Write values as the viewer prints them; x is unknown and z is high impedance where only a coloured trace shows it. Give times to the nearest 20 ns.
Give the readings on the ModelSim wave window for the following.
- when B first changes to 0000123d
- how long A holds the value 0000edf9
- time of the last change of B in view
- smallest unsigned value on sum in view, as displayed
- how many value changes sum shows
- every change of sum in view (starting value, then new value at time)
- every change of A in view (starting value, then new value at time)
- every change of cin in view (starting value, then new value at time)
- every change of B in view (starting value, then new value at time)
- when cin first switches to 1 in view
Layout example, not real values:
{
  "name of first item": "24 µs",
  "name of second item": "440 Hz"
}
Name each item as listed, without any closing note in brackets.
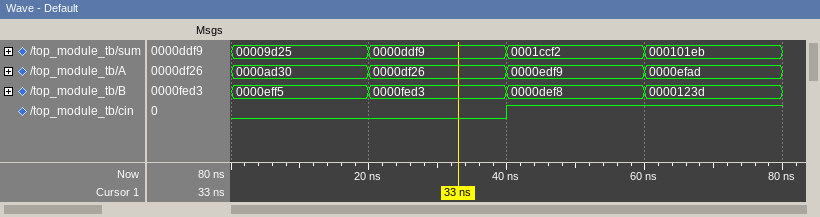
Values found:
{
  "when B first changes to 0000123d": "60 ns",
  "how long A holds the value 0000edf9": "20 ns",
  "time of the last change of B in view": "60 ns",
  "smallest unsigned value on sum in view, as displayed": "00009d25",
  "how many value changes sum shows": "3",
  "every change of sum in view": "00009d25, 0000ddf9 at 20 ns, 0001ccf2 at 40 ns, 000101eb at 60 ns",
  "every change of A in view": "0000ad30, 0000df26 at 20 ns, 0000edf9 at 40 ns, 0000efad at 60 ns",
  "every change of cin in view": "0, 1 at 40 ns",
  "every change of B in view": "0000eff5, 0000fed3 at 20 ns, 0000def8 at 40 ns, 0000123d at 60 ns",
  "when cin first switches to 1 in view": "40 ns"
}
